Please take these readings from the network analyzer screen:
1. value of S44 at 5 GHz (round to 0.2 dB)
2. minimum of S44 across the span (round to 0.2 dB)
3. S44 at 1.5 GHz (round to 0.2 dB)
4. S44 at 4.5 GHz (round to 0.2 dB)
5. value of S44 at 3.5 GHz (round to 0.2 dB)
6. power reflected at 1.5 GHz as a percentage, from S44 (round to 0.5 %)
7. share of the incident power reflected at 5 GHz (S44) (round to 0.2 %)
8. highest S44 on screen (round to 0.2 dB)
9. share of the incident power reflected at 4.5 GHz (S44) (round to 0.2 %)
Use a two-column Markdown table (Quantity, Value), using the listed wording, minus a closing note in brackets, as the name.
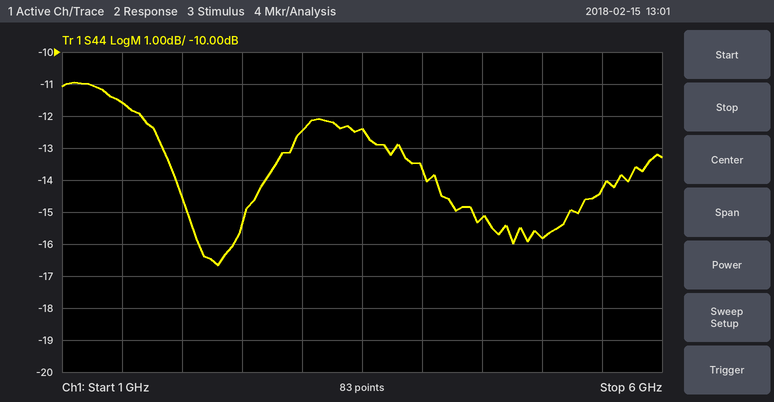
| Quantity | Value |
|---|---|
| value of S44 at 5 GHz | -15.8 dB |
| minimum of S44 across the span | -16.6 dB |
| S44 at 1.5 GHz | -11.6 dB |
| S44 at 4.5 GHz | -15.2 dB |
| value of S44 at 3.5 GHz | -12.4 dB |
| power reflected at 1.5 GHz as a percentage, from S44 | 7.0 % |
| share of the incident power reflected at 5 GHz (S44) | 2.6 % |
| highest S44 on screen | -11.0 dB |
| share of the incident power reflected at 4.5 GHz (S44) | 3.0 % |
